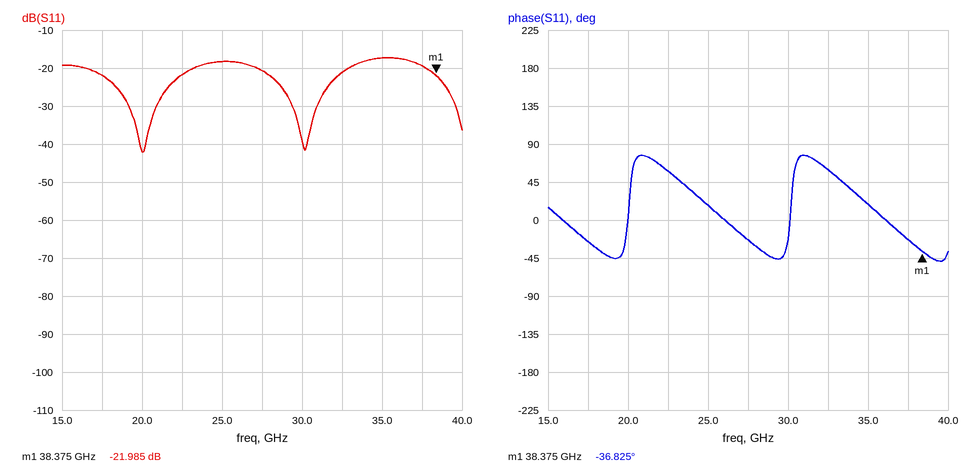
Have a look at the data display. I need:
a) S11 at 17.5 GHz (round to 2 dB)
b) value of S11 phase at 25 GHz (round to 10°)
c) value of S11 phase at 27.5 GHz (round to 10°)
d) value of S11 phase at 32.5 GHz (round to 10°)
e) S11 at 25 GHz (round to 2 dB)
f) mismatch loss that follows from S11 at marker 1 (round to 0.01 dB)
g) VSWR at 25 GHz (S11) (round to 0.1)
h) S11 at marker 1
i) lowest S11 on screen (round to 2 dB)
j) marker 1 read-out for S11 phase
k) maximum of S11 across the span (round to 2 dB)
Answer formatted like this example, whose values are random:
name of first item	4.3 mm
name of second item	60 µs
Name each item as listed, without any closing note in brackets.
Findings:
S11 at 17.5 GHz	-22 dB
value of S11 phase at 25 GHz	20°
value of S11 phase at 27.5 GHz	-20°
value of S11 phase at 32.5 GHz	60°
S11 at 25 GHz	-18 dB
mismatch loss that follows from S11 at marker 1	0.03 dB
VSWR at 25 GHz (S11)	1.3
S11 at marker 1	-21.985 dB
lowest S11 on screen	-42 dB
marker 1 read-out for S11 phase	-36.825°
maximum of S11 across the span	-18 dB
